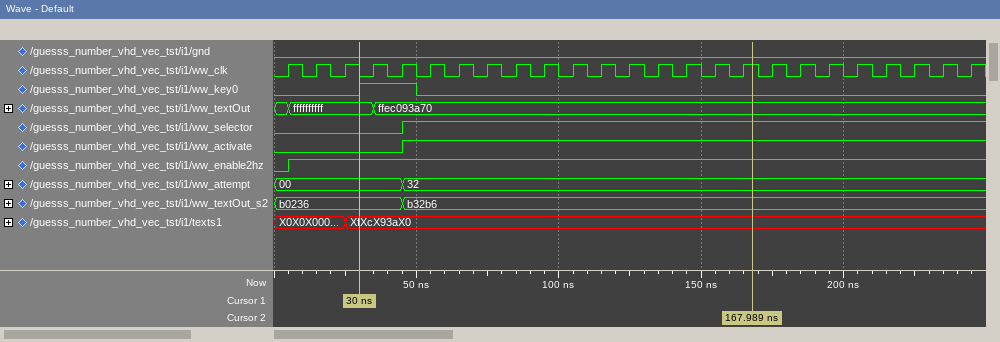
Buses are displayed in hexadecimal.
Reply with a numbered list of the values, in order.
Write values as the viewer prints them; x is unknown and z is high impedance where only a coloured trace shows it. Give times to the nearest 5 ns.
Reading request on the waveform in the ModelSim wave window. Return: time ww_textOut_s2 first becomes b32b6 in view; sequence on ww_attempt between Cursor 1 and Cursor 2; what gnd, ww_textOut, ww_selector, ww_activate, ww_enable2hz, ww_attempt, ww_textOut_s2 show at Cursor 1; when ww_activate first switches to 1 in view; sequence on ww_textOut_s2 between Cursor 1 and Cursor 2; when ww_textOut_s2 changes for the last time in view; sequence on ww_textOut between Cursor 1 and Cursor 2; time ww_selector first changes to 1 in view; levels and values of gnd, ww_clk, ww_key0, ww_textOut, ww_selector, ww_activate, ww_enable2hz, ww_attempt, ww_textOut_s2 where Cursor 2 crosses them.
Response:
1. 45 ns
2. 00, 32
3. gnd=0, ww_textOut=ffffffffff, ww_selector=0, ww_activate=0, ww_enable2hz=1, ww_attempt=00, ww_textOut_s2=b0236
4. 45 ns
5. b0236, b32b6
6. 45 ns
7. ffffffffff, ffec093a70
8. 45 ns
9. gnd=0, ww_clk=1, ww_key0=0, ww_textOut=ffec093a70, ww_selector=1, ww_activate=1, ww_enable2hz=1, ww_attempt=32, ww_textOut_s2=b32b6
